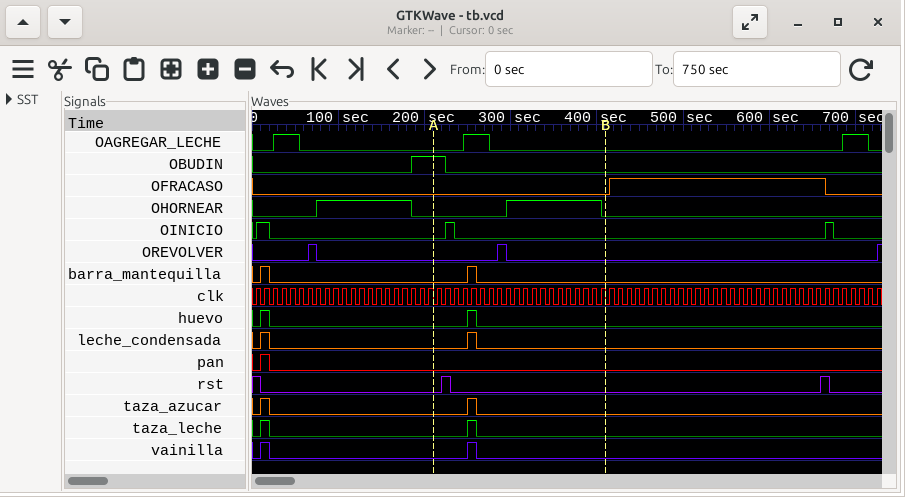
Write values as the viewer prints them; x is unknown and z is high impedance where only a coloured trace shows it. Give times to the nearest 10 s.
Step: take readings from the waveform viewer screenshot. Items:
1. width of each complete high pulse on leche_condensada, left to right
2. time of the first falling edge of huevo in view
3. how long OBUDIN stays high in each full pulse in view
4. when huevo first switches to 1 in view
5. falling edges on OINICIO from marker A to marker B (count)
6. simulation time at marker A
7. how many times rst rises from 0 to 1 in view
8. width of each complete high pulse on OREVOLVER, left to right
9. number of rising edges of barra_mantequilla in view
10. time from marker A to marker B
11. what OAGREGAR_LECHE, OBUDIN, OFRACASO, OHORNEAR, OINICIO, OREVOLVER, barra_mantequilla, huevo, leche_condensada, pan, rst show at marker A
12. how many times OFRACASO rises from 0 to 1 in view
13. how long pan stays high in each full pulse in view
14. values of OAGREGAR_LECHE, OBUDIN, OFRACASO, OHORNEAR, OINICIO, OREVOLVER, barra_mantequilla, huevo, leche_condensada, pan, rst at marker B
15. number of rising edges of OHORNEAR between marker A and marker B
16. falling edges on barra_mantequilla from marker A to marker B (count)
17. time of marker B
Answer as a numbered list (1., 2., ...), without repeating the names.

1. 10 s, 10 s
2. 20 s
3. 40 s
4. 10 s
5. 1
6. 210 s
7. 2
8. 10 s, 10 s
9. 2
10. 200 s
11. OAGREGAR_LECHE=0, OBUDIN=1, OFRACASO=0, OHORNEAR=0, OINICIO=0, OREVOLVER=0, barra_mantequilla=0, huevo=0, leche_condensada=0, pan=0, rst=0
12. 1
13. 10 s
14. OAGREGAR_LECHE=0, OBUDIN=0, OFRACASO=0, OHORNEAR=0, OINICIO=0, OREVOLVER=0, barra_mantequilla=0, huevo=0, leche_condensada=0, pan=0, rst=0
15. 1
16. 1
17. 410 s
